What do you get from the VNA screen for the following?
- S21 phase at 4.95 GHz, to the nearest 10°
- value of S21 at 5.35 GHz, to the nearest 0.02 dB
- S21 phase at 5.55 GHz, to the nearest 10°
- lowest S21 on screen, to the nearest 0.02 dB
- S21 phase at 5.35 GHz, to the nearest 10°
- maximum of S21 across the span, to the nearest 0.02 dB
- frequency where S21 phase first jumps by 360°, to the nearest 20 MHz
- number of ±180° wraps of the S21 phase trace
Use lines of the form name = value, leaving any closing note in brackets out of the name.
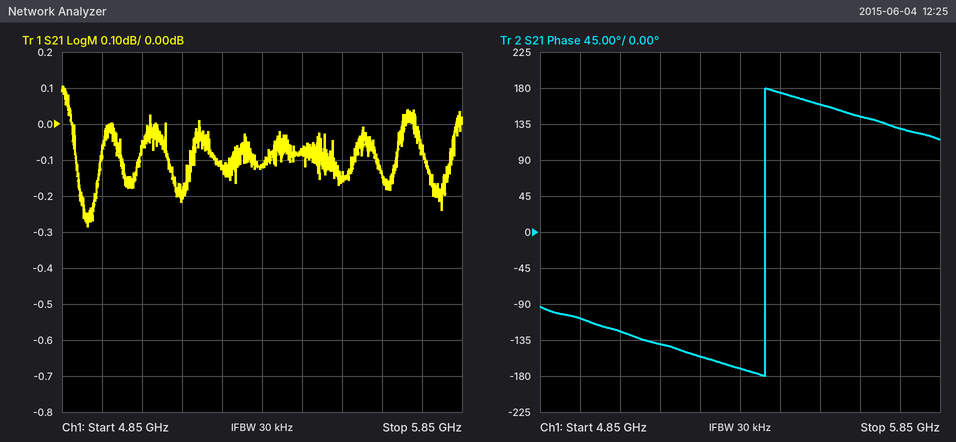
S21 phase at 4.95 GHz, to the nearest 10° = -110°
value of S21 at 5.35 GHz, to the nearest 0.02 dB = -0.12 dB
S21 phase at 5.55 GHz, to the nearest 10° = 160°
lowest S21 on screen, to the nearest 0.02 dB = -0.28 dB
S21 phase at 5.35 GHz, to the nearest 10° = -170°
maximum of S21 across the span, to the nearest 0.02 dB = 0.10 dB
frequency where S21 phase first jumps by 360°, to the nearest 20 MHz = 5.42 GHz
number of ±180° wraps of the S21 phase trace = 1
